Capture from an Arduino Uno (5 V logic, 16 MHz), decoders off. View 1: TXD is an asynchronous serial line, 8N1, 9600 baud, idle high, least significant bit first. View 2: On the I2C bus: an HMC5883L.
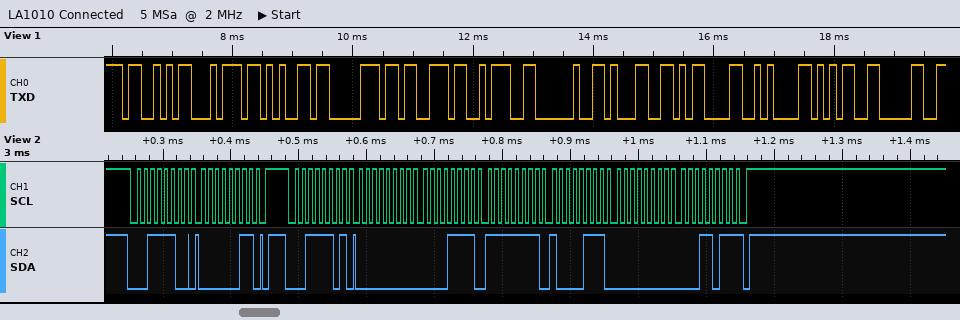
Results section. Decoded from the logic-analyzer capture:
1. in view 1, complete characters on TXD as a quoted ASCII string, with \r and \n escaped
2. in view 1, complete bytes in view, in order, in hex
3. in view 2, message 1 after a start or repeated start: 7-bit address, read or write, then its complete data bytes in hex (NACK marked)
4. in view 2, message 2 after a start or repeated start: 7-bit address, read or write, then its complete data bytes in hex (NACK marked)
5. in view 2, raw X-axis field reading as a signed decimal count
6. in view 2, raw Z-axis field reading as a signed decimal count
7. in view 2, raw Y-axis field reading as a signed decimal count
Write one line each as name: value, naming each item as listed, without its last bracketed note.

in view 1, complete characters on TXD as a quoted ASCII string, with \r and \n escaped: "Steps: 1\r\n50"
in view 1, complete bytes in view, in order, in hex: 0x53 0x74 0x65 0x70 0x73 0x3A 0x20 0x31 0x0D 0x0A 0x35 0x30
in view 2, message 1 after a start or repeated start: 7-bit address, read or write, then its complete data bytes in hex: 0x1E write: 03
in view 2, message 2 after a start or repeated start: 7-bit address, read or write, then its complete data bytes in hex: 0x1E read: 00 0F FF 87 00 1B NACK
in view 2, raw X-axis field reading as a signed decimal count: 15
in view 2, raw Z-axis field reading as a signed decimal count: -121
in view 2, raw Y-axis field reading as a signed decimal count: 27
